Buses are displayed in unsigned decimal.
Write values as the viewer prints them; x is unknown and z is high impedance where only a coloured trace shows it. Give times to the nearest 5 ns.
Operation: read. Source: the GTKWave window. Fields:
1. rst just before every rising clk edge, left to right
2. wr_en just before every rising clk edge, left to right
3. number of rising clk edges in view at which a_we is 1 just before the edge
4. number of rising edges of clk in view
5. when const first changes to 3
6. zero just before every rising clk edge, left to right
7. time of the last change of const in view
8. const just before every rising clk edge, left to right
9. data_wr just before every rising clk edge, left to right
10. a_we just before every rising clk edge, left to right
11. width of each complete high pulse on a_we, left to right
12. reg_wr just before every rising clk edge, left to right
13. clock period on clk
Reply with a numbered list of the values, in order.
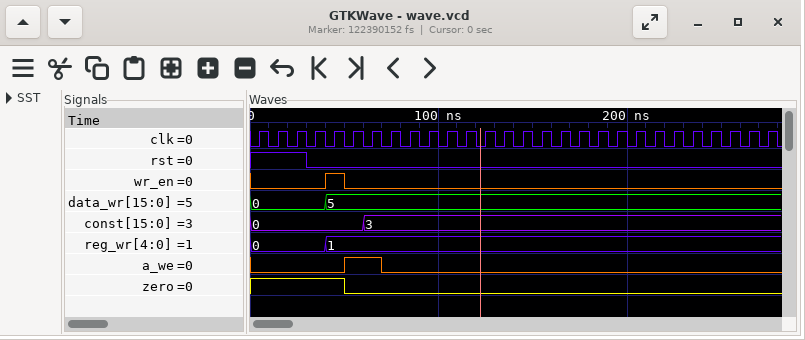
1. 1 1 1 0 0 0 0 0 0 0 0 0 0 0 0 0 0 0 0 0 0 0 0 0 0 0 0 0
2. 0 0 0 0 1 0 0 0 0 0 0 0 0 0 0 0 0 0 0 0 0 0 0 0 0 0 0 0
3. 2
4. 28
5. 60 ns
6. 1 1 1 1 1 0 0 0 0 0 0 0 0 0 0 0 0 0 0 0 0 0 0 0 0 0 0 0
7. 60 ns
8. 0, 0, 0, 0, 0, 0, 3, 3, 3, 3, 3, 3, 3, 3, 3, 3, 3, 3, 3, 3, 3, 3, 3, 3, 3, 3, 3, 3
9. 0, 0, 0, 0, 5, 5, 5, 5, 5, 5, 5, 5, 5, 5, 5, 5, 5, 5, 5, 5, 5, 5, 5, 5, 5, 5, 5, 5
10. 0 0 0 0 0 1 1 0 0 0 0 0 0 0 0 0 0 0 0 0 0 0 0 0 0 0 0 0
11. 20 ns
12. 0, 0, 0, 0, 1, 1, 1, 1, 1, 1, 1, 1, 1, 1, 1, 1, 1, 1, 1, 1, 1, 1, 1, 1, 1, 1, 1, 1
13. 10 ns
